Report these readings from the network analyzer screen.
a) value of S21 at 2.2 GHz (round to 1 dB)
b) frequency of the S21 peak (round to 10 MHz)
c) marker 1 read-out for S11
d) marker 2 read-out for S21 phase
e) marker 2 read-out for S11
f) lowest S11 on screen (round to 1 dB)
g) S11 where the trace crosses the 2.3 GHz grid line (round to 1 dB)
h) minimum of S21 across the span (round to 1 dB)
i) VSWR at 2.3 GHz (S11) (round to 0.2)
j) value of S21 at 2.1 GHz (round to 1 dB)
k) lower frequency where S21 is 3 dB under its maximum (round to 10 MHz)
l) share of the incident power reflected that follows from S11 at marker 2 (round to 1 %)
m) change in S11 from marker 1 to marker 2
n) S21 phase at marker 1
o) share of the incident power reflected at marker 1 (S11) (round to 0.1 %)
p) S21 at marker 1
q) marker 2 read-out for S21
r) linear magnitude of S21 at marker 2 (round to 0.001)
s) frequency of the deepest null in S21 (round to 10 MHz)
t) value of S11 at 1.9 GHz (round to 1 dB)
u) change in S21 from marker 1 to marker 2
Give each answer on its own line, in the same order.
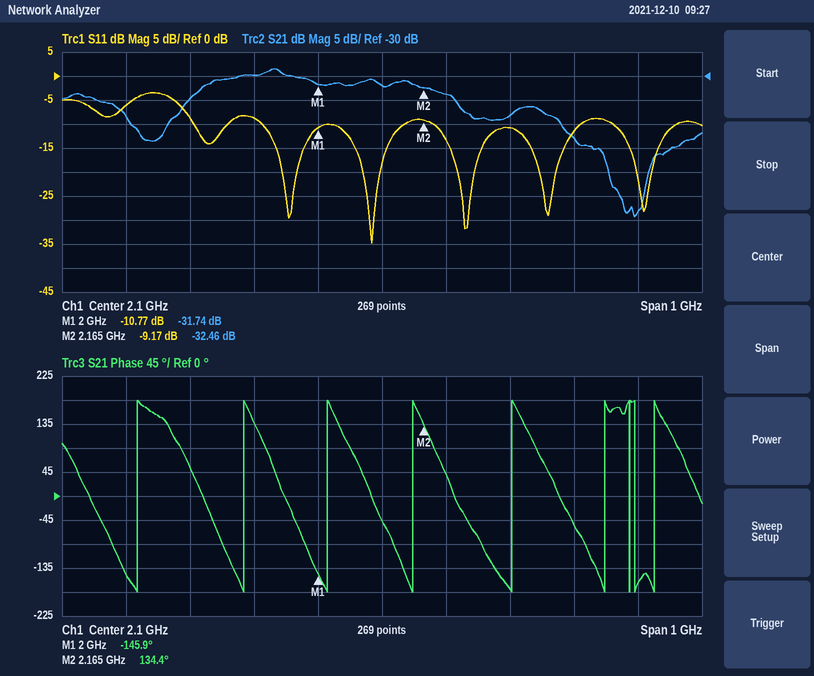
-34 dB
1.93 GHz
-10.77 dB
134.4°
-9.17 dB
-35 dB
-11 dB
-59 dB
1.8
-32 dB
1.83 GHz
12 %
1.60 dB
-145.9°
8.4 %
-31.74 dB
-32.46 dB
0.024
2.49 GHz
-9 dB
-0.72 dB
